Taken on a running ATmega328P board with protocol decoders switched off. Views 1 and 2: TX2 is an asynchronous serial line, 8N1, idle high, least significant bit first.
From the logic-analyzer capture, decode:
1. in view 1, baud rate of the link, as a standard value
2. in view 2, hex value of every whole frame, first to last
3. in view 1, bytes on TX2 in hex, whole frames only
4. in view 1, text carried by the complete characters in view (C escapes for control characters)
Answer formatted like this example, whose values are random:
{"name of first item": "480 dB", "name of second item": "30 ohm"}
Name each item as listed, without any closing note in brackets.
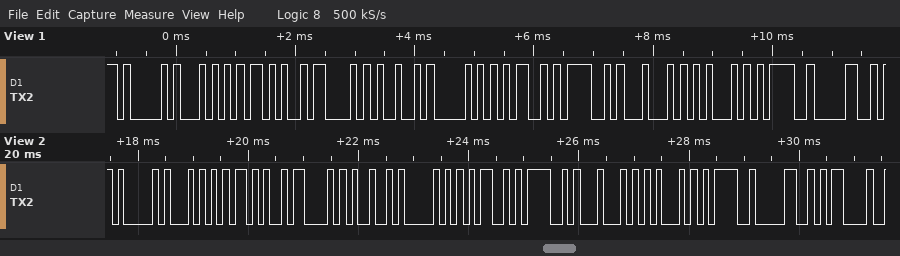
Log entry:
{"in view 1, baud rate of the link, as a standard value": "9600 baud", "in view 2, hex value of every whole frame, first to last": "0x41 0x54 0x2B 0x43 0x49 0x50 0x4D 0x4F 0x44 0x45 0x3D 0x30 0x0D", "in view 1, bytes on TX2 in hex, whole frames only": "41 54 2B 43 49 50 4D 4F 44 45 3D 30", "in view 1, text carried by the complete characters in view": "\"AT+CIPMODE=0\""}
